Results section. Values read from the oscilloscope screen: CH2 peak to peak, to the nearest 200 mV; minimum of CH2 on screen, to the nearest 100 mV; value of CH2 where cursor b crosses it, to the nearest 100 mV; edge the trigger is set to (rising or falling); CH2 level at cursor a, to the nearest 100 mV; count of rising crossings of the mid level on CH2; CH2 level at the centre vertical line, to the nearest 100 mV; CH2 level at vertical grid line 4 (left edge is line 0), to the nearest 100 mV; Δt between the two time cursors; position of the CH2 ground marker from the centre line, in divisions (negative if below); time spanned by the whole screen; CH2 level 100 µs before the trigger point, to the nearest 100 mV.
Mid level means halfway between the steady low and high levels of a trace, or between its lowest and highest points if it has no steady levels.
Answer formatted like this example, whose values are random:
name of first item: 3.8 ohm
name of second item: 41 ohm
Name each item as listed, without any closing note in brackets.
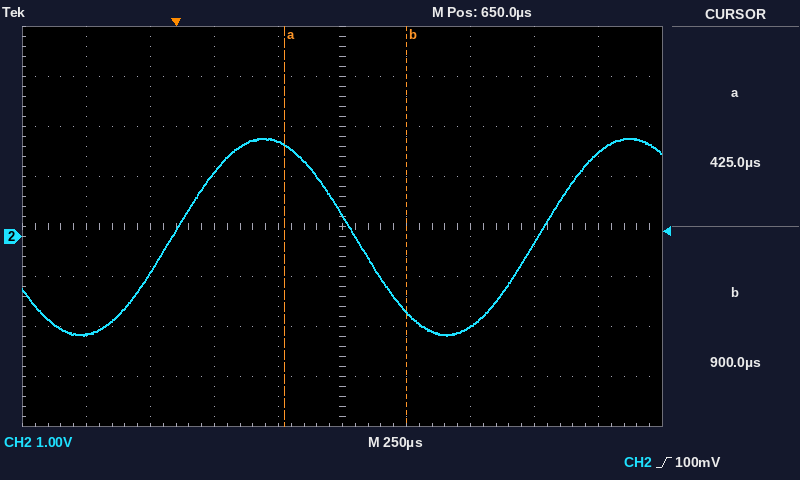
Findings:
CH2 peak to peak, to the nearest 200 mV: 4.0 V
minimum of CH2 on screen, to the nearest 100 mV: -2.0 V
value of CH2 where cursor b crosses it, to the nearest 100 mV: -1.5 V
edge the trigger is set to: rising
CH2 level at cursor a, to the nearest 100 mV: 1.8 V
count of rising crossings of the mid level on CH2: 2
CH2 level at the centre vertical line, to the nearest 100 mV: 400 mV
CH2 level at vertical grid line 4 (left edge is line 0), to the nearest 100 mV: 1.9 V
Δt between the two time cursors: 475 µs
position of the CH2 ground marker from the centre line, in divisions: -0.2 div
time spanned by the whole screen: 2.5 ms
CH2 level 100 µs before the trigger point, to the nearest 100 mV: -700 mV
